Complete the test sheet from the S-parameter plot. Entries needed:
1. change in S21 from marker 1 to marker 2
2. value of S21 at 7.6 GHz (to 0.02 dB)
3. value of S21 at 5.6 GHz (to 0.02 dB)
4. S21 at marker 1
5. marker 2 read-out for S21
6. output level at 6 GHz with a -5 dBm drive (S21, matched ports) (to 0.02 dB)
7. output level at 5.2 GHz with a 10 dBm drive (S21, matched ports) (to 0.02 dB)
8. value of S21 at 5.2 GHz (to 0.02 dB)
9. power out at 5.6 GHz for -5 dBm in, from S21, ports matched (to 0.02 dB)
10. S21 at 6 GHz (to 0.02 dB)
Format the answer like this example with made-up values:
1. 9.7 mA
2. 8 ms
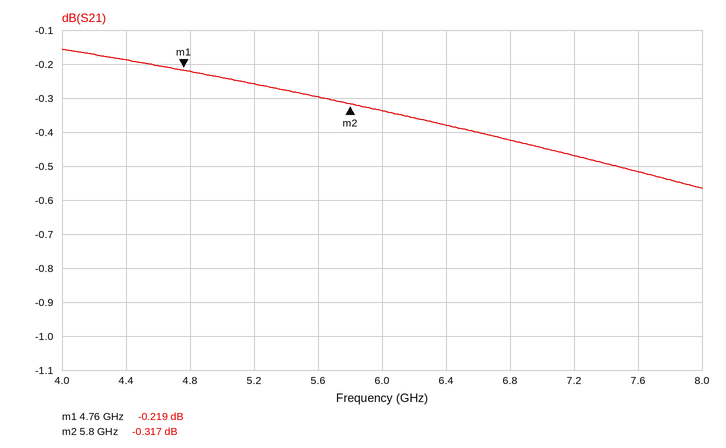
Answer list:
1. -0.098 dB
2. -0.52 dB
3. -0.30 dB
4. -0.219 dB
5. -0.317 dB
6. -5.34 dBm
7. 9.74 dBm
8. -0.26 dB
9. -5.30 dBm
10. -0.34 dB
